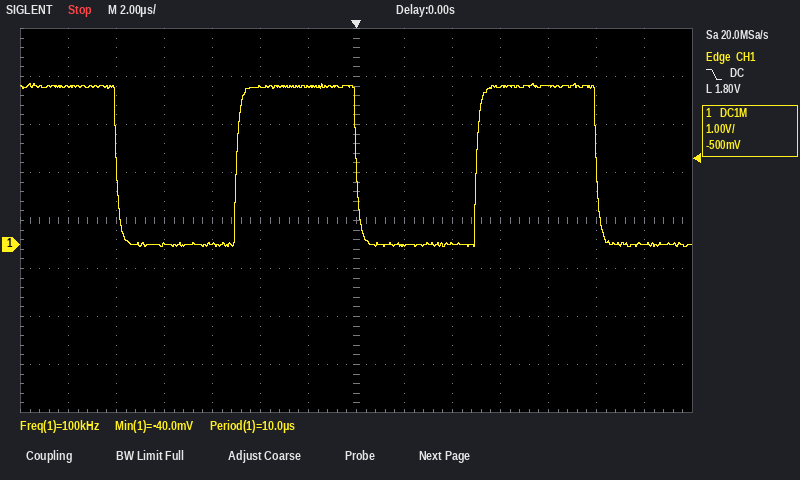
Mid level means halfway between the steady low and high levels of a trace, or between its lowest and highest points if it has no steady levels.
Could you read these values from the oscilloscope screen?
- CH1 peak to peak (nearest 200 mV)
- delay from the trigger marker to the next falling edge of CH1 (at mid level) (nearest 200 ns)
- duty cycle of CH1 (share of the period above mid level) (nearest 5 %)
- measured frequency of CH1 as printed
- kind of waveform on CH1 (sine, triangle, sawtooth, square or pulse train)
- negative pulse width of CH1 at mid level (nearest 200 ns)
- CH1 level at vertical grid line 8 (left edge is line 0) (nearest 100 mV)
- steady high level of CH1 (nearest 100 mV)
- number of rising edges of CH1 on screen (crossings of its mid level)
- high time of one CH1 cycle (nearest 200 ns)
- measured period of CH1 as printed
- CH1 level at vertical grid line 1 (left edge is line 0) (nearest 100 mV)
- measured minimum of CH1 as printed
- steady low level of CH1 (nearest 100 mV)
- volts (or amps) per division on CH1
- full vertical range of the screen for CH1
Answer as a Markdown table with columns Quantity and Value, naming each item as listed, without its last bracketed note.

| Quantity | Value |
|---|---|
| CH1 peak to peak | 3.4 V |
| delay from the trigger marker to the next falling edge of CH1 (at mid level) | 10.0 µs |
| duty cycle of CH1 (share of the period above mid level) | 50 % |
| measured frequency of CH1 as printed | 100 kHz |
| kind of waveform on CH1 | square |
| negative pulse width of CH1 at mid level | 5.0 µs |
| CH1 level at vertical grid line 8 (left edge is line 0) | 0.0 V |
| steady high level of CH1 | 3.3 V |
| number of rising edges of CH1 on screen | 2 |
| high time of one CH1 cycle | 5.0 µs |
| measured period of CH1 as printed | 10.0 µs |
| CH1 level at vertical grid line 1 (left edge is line 0) | 3.3 V |
| measured minimum of CH1 as printed | -40.0 mV |
| steady low level of CH1 | 0.0 V |
| volts (or amps) per division on CH1 | 1 V |
| full vertical range of the screen for CH1 | 8 V |
